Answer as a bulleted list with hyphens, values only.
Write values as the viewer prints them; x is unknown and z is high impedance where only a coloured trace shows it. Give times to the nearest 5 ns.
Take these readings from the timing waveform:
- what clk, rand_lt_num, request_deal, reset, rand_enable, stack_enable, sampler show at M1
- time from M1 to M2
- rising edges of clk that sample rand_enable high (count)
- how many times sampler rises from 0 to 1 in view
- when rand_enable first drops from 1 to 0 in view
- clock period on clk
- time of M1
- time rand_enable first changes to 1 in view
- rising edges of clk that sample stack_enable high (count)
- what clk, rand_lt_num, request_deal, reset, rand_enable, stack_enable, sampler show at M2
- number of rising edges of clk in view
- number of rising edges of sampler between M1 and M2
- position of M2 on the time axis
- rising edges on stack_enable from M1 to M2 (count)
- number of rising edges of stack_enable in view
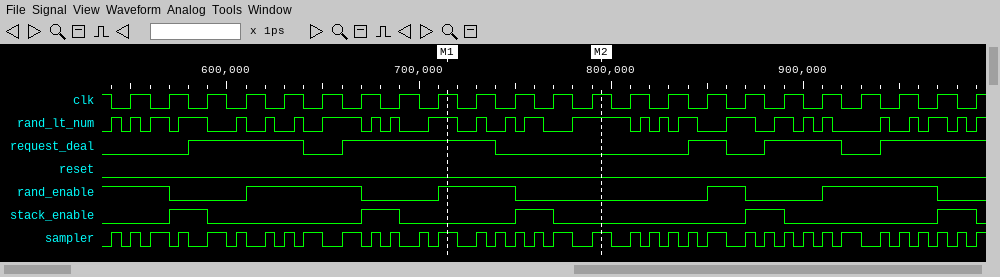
- clk=1, rand_lt_num=1, request_deal=1, reset=0, rand_enable=1, stack_enable=0, sampler=1
- 80 ns
- 11
- 37
- 570 ns
- 20 ns
- 715 ns
- 610 ns
- 5
- clk=1, rand_lt_num=1, request_deal=0, reset=0, rand_enable=0, stack_enable=0, sampler=1
- 23
- 6
- 795 ns
- 1
- 5
